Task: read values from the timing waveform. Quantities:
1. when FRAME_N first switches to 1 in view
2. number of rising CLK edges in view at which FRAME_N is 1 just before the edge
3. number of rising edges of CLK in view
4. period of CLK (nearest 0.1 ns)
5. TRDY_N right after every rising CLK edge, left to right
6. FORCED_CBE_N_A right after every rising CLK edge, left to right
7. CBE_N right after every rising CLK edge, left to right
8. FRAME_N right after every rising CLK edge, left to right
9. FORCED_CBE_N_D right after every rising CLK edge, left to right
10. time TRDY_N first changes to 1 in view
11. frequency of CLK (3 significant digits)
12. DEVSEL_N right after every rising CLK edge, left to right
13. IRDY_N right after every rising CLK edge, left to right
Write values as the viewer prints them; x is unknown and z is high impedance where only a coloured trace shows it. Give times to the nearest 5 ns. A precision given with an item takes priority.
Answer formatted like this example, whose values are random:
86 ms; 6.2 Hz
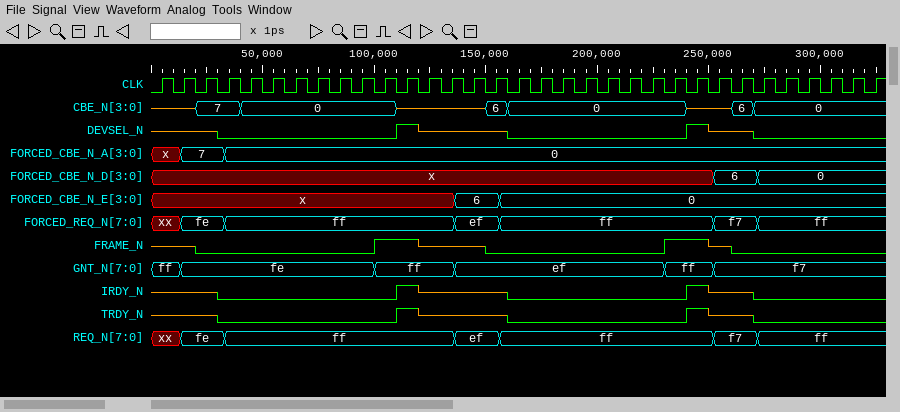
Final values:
100 ns; 4; 33; 10 ns; z z z 0 0 0 0 0 0 0 0 1 z z z z 0 0 0 0 0 0 0 0 1 z z 0 0 0 0 0 0; x, 7, 7, 0, 0, 0, 0, 0, 0, 0, 0, 0, 0, 0, 0, 0, 0, 0, 0, 0, 0, 0, 0, 0, 0, 0, 0, 0, 0, 0, 0, 0, 0; z, z, 7, 7, 0, 0, 0, 0, 0, 0, 0, z, z, z, z, 6, 0, 0, 0, 0, 0, 0, 0, 0, z, z, 6, 0, 0, 0, 0, 0, 0; z z 0 0 0 0 0 0 0 0 1 1 z z z 0 0 0 0 0 0 0 0 1 1 z 0 0 0 0 0 0 0; x, x, x, x, x, x, x, x, x, x, x, x, x, x, x, x, x, x, x, x, x, x, x, x, x, 6, 6, 0, 0, 0, 0, 0, 0; 110 ns; 100 MHz; z z z 0 0 0 0 0 0 0 0 1 z z z z 0 0 0 0 0 0 0 0 1 z z 0 0 0 0 0 0; z z z 0 0 0 0 0 0 0 0 1 z z z z 0 0 0 0 0 0 0 0 1 z z 0 0 0 0 0 0
